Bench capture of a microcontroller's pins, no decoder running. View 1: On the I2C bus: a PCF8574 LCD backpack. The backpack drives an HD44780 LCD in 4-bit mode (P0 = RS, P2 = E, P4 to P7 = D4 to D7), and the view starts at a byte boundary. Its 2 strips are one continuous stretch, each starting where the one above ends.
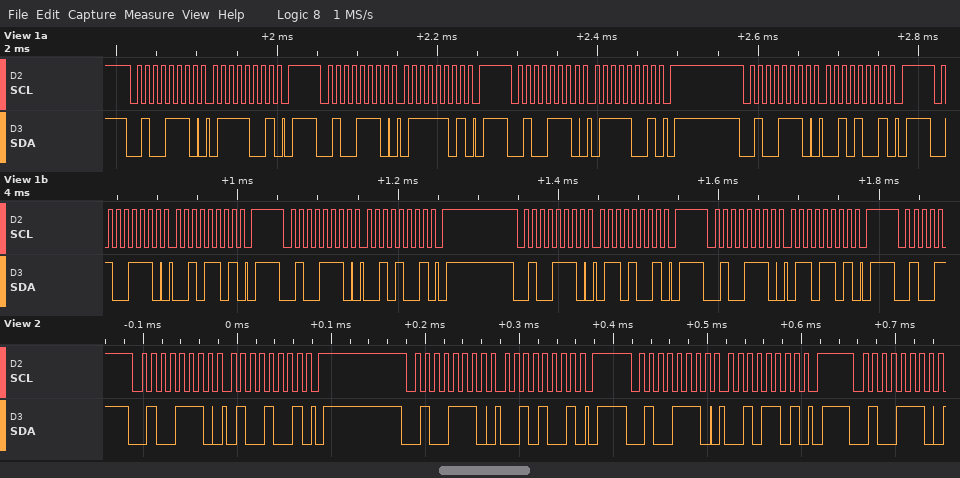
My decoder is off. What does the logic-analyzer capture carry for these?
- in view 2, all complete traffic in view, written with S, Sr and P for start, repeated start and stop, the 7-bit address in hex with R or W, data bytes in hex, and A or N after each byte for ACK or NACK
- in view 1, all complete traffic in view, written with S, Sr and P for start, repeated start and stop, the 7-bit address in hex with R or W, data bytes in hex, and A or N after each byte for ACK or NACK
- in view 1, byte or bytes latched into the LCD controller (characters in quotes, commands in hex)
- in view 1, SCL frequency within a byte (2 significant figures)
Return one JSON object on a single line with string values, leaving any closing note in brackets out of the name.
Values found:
{"in view 2, all complete traffic in view, written with S, Sr and P for start, repeated start and stop, the 7-bit address in hex with R or W, data bytes in hex, and A or N after each byte for ACK or NACK": "S 27W A 49 A P S 27W A 29 A P S 27W A 2D A P S 27W A", "in view 1, all complete traffic in view, written with S, Sr and P for start, repeated start and stop, the 7-bit address in hex with R or W, data bytes in hex, and A or N after each byte for ACK or NACK": "S 27W A 79 A P S 27W A 7D A P S 27W A 79 A P S 27W A 29 A P S 27W A 2D A P S 27W A 29 A P S 27W A 69 A P S 27W A 6D A P", "in view 1, byte or bytes latched into the LCD controller": "'r'", "in view 1, SCL frequency within a byte": "100 kHz"}
